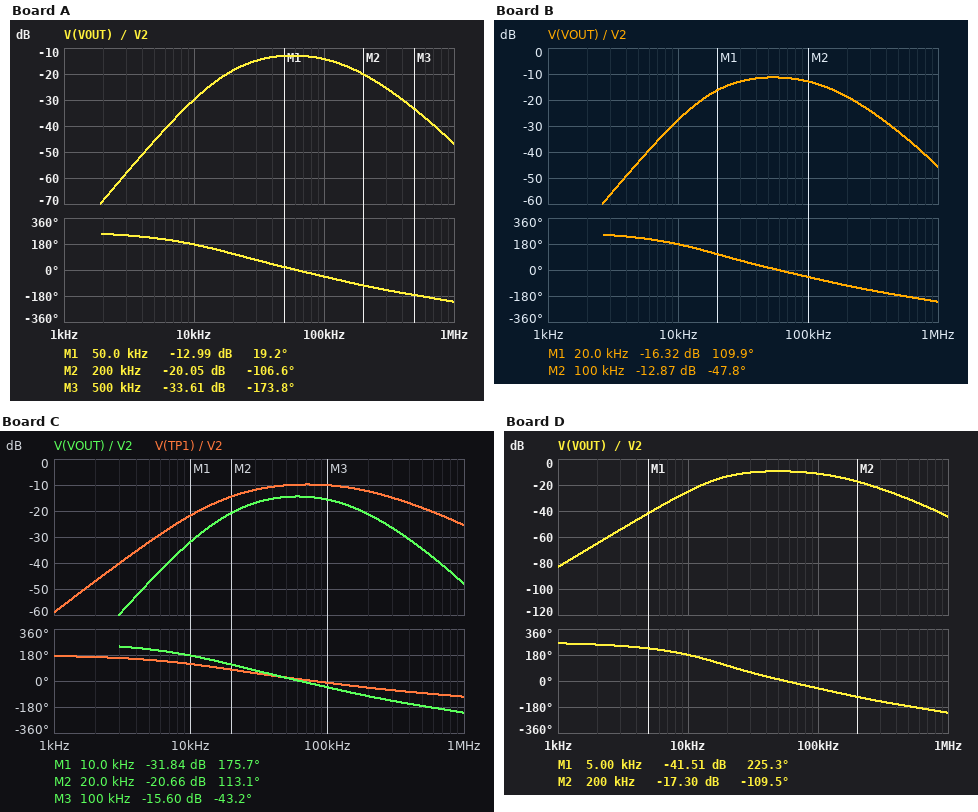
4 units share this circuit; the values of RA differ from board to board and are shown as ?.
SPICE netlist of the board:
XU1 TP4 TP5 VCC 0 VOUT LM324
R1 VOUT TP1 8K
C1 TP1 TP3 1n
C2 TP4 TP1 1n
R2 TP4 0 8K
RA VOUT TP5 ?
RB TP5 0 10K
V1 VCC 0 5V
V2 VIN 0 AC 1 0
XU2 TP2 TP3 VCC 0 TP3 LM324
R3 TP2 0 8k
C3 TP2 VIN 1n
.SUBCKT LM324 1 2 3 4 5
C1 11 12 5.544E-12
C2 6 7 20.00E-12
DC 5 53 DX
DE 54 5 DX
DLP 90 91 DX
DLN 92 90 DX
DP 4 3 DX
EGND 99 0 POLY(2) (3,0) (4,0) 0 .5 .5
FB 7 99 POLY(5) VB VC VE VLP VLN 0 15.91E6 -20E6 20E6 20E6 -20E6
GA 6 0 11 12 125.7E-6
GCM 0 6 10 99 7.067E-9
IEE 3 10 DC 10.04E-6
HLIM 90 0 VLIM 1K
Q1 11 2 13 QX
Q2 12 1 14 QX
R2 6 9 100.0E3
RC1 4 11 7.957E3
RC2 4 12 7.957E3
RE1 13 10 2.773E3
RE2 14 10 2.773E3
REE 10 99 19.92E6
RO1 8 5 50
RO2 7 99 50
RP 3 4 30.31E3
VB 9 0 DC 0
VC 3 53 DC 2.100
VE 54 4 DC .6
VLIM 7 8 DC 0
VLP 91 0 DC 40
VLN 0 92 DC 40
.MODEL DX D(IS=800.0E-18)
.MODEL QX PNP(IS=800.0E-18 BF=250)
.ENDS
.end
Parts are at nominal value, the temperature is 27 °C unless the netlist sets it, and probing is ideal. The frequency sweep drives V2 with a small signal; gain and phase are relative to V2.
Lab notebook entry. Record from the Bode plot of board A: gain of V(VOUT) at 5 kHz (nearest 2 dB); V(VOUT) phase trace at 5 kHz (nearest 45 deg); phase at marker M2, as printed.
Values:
-46 dB
225 deg
-106.6 deg
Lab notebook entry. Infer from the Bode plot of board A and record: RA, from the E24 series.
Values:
12 kΩ
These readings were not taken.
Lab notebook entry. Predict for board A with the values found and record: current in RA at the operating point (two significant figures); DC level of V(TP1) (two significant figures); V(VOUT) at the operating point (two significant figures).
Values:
1.9 µA
42 mV
42 mV
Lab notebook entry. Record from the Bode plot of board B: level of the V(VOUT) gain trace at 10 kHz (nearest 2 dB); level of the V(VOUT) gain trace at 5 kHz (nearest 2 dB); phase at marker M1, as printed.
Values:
-28 dB
-44 dB
109.9 deg
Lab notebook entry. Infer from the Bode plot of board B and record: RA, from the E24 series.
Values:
18 kΩ
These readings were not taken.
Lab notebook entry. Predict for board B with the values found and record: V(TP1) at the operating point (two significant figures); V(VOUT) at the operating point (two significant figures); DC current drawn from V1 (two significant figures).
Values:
46 mV
46 mV
350 µA
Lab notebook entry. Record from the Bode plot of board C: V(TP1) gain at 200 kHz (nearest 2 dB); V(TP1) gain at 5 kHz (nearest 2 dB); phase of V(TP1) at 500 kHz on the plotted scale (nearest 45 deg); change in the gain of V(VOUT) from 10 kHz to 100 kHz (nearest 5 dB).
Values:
-12 dB
-32 dB
-90 deg
15 dB
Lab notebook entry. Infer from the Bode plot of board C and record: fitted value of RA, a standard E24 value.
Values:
7.5 kΩ
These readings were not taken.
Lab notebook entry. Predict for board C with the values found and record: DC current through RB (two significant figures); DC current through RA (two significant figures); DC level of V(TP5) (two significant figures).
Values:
2.2 µA
2.2 µA
22 mV
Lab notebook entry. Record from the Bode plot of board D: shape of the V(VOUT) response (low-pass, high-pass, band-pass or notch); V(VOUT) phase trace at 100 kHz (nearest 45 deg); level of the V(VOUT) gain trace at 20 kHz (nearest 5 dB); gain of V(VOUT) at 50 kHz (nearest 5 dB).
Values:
band-pass
-45 deg
-15 dB
-10 dB
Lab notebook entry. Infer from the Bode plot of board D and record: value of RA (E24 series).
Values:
27 kΩ
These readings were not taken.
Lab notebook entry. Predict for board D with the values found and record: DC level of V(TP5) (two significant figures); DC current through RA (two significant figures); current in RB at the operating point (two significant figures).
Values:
14 mV
1.4 µA
1.4 µA
